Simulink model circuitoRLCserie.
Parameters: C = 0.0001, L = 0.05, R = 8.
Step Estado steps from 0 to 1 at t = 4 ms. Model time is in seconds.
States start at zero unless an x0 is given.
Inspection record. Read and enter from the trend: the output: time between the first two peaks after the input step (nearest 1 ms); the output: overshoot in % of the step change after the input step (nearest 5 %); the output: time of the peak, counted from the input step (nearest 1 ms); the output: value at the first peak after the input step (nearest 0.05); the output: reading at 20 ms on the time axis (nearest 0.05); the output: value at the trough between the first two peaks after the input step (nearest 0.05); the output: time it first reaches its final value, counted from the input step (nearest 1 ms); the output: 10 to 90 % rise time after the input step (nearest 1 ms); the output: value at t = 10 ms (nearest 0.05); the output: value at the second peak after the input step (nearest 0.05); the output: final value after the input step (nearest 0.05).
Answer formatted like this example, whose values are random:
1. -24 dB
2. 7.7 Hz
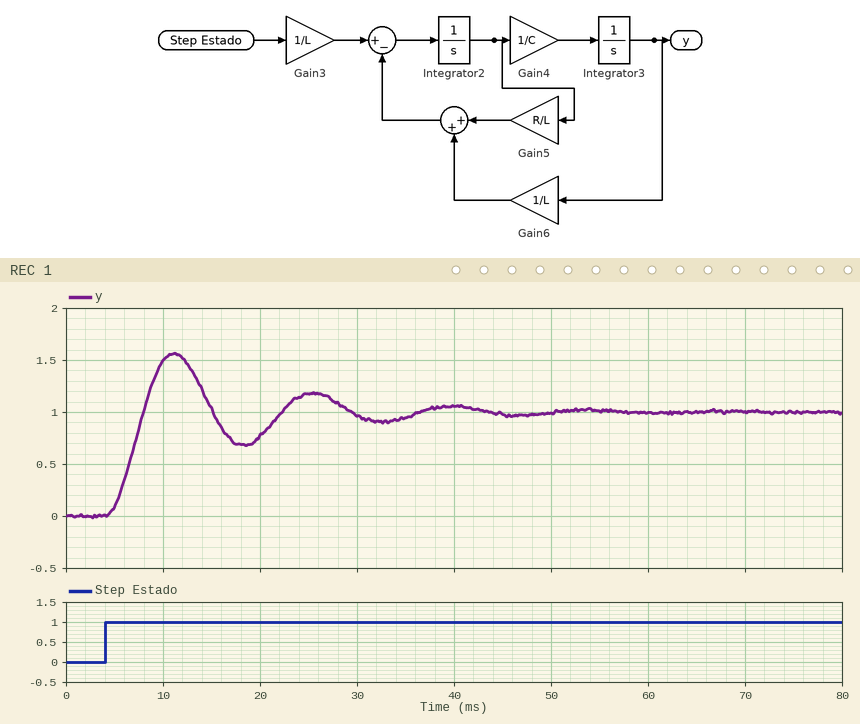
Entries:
1. 14 ms
2. 55 %
3. 7 ms
4. 1.55
5. 0.75
6. 0.70
7. 4 ms
8. 3 ms
9. 1.50
10. 1.20
11. 1.00
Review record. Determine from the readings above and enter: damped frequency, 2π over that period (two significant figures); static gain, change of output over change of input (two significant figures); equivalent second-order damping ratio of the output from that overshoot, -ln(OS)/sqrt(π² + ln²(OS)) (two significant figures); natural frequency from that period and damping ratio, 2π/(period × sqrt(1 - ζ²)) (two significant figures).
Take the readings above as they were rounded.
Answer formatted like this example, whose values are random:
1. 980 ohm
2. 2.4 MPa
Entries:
1. 0.45 rad/ms
2. 1.0
3. 0.19
4. 0.46 rad/ms
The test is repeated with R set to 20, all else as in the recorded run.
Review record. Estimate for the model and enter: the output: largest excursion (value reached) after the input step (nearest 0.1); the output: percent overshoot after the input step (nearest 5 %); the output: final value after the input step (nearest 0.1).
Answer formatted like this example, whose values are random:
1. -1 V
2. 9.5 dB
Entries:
1. 1.2
2. 20 %
3. 1.0
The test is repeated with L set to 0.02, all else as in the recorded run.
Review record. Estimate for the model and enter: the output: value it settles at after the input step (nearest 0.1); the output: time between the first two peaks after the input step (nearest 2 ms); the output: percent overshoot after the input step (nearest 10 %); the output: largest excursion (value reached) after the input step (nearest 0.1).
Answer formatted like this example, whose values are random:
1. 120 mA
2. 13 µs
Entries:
1. 1.0
2. 10 ms
3. 40 %
4. 1.4
